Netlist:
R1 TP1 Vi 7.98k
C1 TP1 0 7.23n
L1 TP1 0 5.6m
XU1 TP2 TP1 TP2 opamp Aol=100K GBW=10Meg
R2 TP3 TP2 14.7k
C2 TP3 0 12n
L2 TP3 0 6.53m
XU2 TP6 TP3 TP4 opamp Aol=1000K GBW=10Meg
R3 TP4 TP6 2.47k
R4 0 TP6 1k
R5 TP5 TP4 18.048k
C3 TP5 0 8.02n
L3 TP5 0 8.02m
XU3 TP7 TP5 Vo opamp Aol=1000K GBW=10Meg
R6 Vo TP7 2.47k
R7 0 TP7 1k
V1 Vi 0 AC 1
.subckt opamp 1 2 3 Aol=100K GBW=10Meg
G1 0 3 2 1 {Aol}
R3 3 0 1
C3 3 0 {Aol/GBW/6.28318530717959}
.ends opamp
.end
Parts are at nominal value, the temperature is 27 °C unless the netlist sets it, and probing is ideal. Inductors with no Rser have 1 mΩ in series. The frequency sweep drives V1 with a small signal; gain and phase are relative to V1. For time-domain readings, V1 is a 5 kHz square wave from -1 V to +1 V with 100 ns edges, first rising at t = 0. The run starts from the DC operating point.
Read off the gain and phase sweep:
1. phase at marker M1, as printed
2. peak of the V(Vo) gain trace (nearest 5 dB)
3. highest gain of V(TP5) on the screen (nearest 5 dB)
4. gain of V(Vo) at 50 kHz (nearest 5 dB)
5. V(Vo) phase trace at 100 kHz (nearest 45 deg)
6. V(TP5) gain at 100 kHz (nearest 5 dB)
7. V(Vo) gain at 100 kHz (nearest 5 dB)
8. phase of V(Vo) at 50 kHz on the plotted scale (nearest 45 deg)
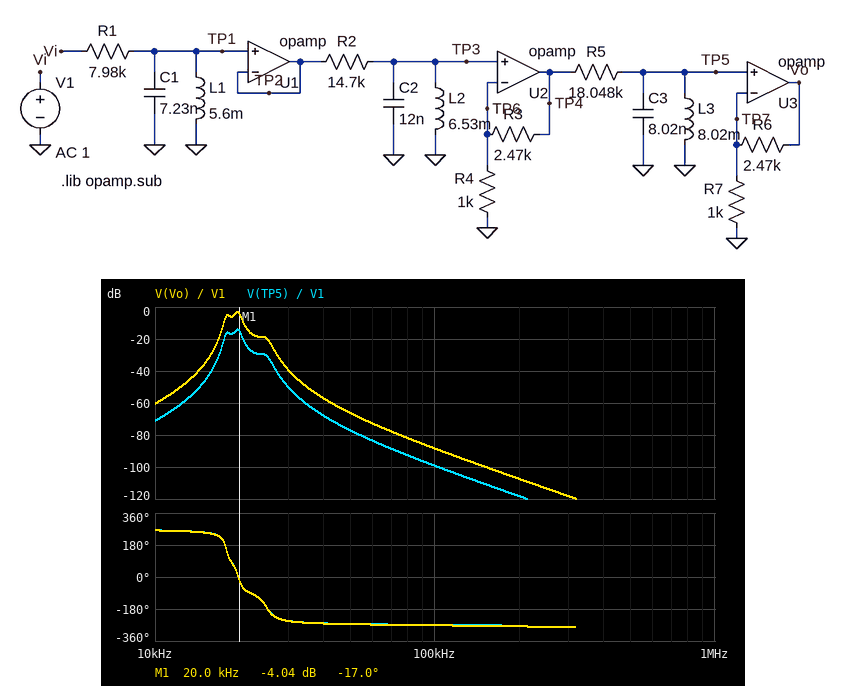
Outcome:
-17.0 deg
-5 dB
-15 dB
-65 dB
-270 deg
-100 dB
-90 dB
-270 deg
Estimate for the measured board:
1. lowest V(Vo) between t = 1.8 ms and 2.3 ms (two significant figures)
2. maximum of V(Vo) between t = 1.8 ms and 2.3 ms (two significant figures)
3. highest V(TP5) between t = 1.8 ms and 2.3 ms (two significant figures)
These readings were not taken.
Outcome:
-34 mV
34 mV
9.7 mV
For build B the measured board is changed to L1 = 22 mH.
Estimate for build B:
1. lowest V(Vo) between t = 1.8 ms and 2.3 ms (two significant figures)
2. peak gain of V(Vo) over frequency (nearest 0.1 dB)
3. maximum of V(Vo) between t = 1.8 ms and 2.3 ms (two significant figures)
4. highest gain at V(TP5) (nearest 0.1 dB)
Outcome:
-40 mV
-0.4 dB
40 mV
-11.2 dB
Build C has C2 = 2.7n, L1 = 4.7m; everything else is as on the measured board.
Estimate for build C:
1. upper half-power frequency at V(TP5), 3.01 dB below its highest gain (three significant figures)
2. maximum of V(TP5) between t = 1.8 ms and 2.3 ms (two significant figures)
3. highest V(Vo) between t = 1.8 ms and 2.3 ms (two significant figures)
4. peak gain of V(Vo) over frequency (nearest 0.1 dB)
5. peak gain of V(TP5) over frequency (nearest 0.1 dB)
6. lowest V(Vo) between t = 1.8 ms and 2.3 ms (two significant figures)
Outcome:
28.8 kHz
10 mV
36 mV
-15.9 dB
-26.7 dB
-36 mV
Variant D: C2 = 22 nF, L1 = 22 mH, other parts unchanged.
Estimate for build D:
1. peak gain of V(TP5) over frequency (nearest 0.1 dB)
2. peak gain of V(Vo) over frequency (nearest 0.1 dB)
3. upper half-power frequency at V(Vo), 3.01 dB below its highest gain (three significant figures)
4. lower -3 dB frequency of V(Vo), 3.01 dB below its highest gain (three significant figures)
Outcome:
-13.5 dB
-2.7 dB
13.5 kHz
13.0 kHz
